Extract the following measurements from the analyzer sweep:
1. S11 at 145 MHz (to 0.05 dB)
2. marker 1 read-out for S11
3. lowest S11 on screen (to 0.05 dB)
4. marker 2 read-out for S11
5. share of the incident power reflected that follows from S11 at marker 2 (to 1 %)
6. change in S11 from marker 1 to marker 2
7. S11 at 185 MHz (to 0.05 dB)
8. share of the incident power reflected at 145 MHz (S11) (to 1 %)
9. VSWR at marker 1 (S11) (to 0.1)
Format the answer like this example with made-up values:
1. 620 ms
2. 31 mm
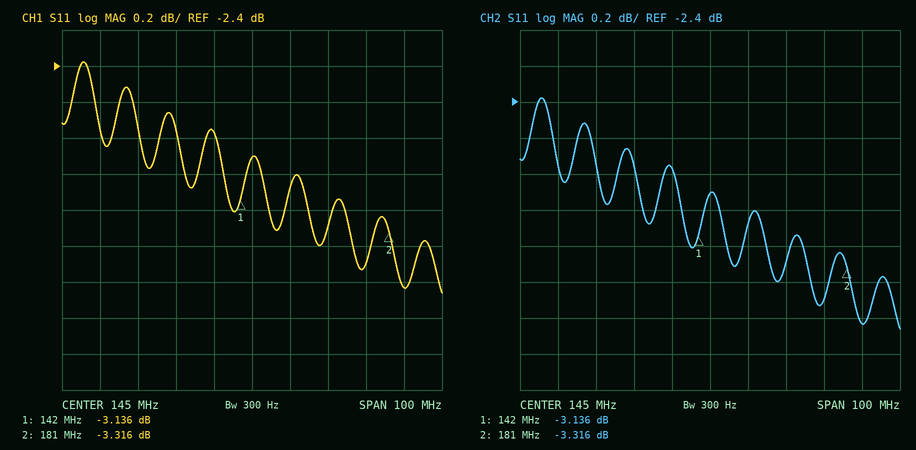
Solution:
1. -2.90 dB
2. -3.136 dB
3. -3.65 dB
4. -3.316 dB
5. 47 %
6. -0.180 dB
7. -3.65 dB
8. 51 %
9. 5.6
